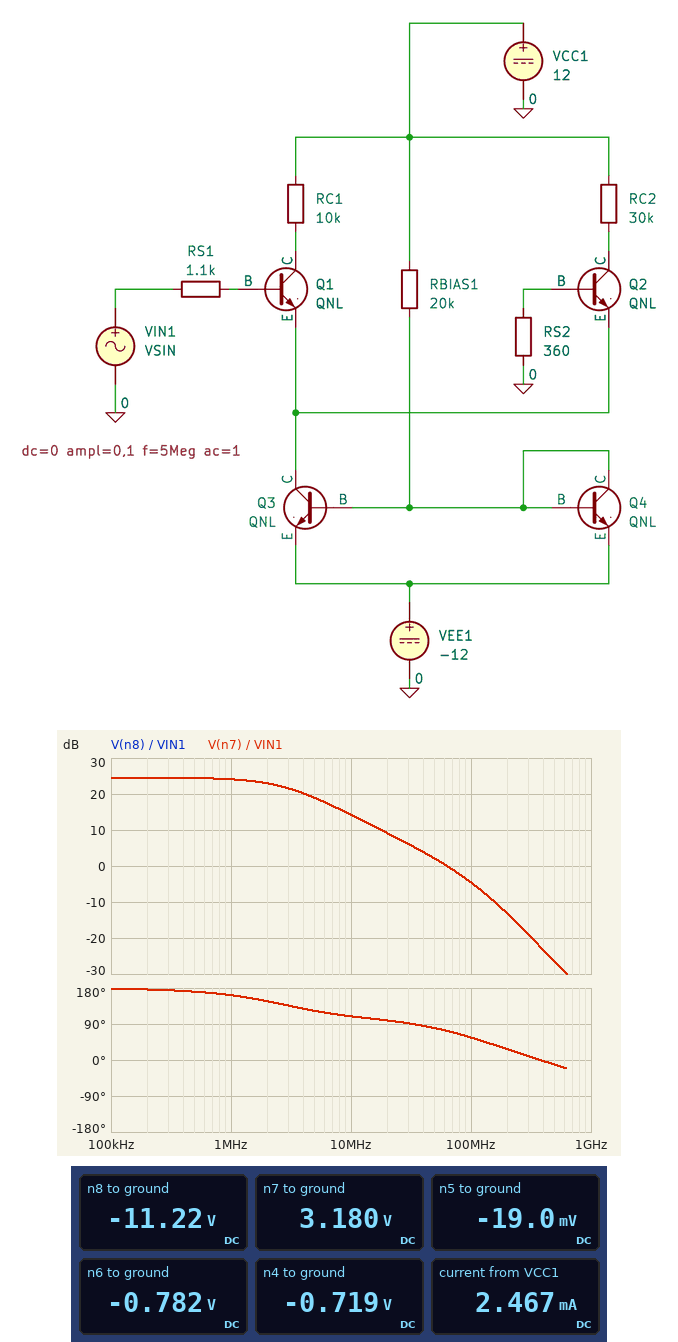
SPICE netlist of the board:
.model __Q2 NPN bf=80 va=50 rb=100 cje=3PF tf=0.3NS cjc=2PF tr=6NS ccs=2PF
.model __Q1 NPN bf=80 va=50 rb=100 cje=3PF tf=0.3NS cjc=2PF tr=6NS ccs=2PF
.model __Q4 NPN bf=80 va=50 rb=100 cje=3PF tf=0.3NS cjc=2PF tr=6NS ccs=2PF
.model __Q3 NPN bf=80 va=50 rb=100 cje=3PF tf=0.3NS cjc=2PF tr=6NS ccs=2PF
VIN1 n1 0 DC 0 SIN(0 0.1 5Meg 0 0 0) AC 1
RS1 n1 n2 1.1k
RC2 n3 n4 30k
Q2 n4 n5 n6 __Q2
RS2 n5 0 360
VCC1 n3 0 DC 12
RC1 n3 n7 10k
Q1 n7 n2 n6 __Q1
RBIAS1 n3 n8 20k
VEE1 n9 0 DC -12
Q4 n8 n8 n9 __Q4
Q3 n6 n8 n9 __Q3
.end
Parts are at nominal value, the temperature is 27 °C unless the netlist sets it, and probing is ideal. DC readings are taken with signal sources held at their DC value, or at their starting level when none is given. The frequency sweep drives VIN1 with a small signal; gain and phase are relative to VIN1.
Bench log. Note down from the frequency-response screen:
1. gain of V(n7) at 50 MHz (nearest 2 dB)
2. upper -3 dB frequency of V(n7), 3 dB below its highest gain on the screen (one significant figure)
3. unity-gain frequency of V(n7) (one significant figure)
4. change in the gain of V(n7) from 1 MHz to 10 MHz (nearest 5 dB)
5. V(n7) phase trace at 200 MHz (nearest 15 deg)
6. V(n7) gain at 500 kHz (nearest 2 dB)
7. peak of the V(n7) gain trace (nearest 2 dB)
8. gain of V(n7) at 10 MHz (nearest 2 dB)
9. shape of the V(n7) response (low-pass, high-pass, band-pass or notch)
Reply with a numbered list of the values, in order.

1. 2 dB
2. 3 MHz
3. 60 MHz
4. -10 dB
5. 30 deg
6. 24 dB
7. 24 dB
8. 14 dB
9. low-pass
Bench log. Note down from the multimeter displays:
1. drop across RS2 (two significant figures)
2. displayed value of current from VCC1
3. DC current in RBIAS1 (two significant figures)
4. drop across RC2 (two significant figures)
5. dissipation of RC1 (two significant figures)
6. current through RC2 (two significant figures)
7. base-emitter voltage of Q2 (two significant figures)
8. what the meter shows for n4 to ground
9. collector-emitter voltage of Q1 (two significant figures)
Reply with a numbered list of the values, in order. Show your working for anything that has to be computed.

1. 0 V - (-19 mV) = 19 mV
2. 2.467 mA
3. (12 V - (-11.22 V)) / 20 kΩ = 1.2 mA
4. 12 V - (-719 mV) = 13 V
5. (12 V - 3.18 V)^2 / 10 kΩ = 7.8 mW
6. (12 V - (-719 mV)) / 30 kΩ = 420 µA
7. -19 mV - (-782 mV) = 760 mV
8. -0.719 V
9. 3.18 V - (-782 mV) = 4.0 V
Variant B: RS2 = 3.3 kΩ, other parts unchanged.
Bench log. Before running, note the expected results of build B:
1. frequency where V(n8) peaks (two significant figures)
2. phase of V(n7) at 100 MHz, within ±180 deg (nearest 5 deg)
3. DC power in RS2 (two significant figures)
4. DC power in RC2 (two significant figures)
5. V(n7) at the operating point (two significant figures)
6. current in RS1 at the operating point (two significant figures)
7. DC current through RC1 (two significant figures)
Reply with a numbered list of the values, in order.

1. 100 MHz
2. 60 deg
3. 280 nW
4. 5.3 mW
5. 2.7 V
6. 11 µA
7. 930 µA
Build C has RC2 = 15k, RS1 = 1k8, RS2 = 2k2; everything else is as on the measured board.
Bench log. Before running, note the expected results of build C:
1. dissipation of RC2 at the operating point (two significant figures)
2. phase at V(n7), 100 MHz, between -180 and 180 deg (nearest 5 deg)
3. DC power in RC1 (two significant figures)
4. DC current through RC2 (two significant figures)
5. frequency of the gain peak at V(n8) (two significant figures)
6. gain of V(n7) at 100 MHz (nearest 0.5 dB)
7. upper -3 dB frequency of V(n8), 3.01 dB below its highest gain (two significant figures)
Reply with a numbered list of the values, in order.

1. 6.1 mW
2. 50 deg
3. 5.1 mW
4. 640 µA
5. 95 MHz
6. -8.0 dB
7. 240 MHz
